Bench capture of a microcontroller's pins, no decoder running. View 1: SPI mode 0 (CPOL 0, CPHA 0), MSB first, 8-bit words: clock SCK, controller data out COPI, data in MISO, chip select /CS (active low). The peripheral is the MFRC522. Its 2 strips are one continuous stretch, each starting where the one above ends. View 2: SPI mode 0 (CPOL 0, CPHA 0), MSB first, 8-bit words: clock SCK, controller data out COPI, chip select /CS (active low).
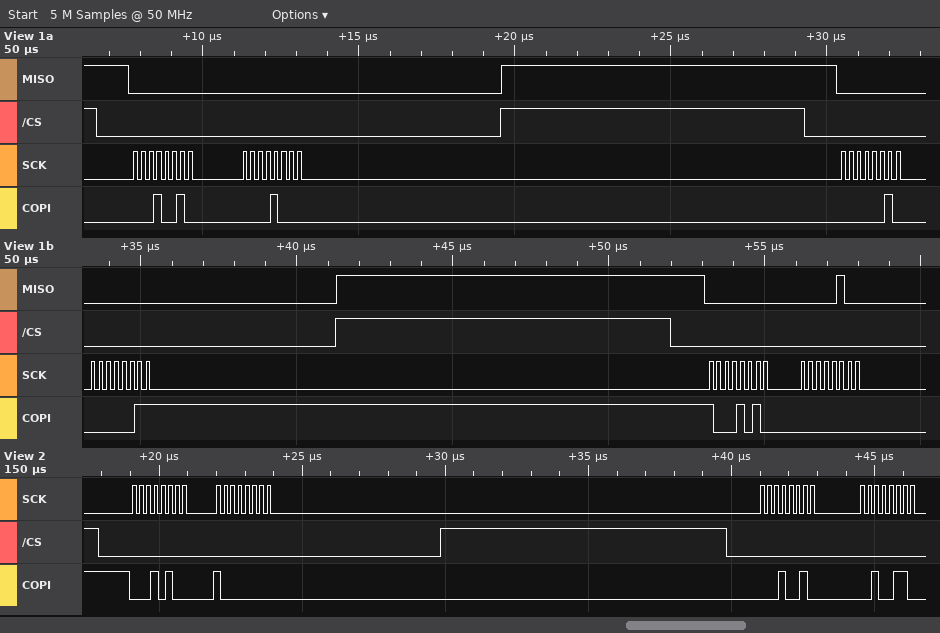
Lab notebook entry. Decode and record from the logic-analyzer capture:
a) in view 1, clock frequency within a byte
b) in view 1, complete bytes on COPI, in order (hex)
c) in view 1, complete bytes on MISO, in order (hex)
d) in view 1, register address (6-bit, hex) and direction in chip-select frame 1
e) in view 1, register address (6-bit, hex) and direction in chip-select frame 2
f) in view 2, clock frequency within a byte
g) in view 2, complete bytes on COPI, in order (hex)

4 MHz
12 08 02 03 8A 00
00 00 00 00 00 04
0x09 write
0x01 write
4 MHz
14 80 12 26
